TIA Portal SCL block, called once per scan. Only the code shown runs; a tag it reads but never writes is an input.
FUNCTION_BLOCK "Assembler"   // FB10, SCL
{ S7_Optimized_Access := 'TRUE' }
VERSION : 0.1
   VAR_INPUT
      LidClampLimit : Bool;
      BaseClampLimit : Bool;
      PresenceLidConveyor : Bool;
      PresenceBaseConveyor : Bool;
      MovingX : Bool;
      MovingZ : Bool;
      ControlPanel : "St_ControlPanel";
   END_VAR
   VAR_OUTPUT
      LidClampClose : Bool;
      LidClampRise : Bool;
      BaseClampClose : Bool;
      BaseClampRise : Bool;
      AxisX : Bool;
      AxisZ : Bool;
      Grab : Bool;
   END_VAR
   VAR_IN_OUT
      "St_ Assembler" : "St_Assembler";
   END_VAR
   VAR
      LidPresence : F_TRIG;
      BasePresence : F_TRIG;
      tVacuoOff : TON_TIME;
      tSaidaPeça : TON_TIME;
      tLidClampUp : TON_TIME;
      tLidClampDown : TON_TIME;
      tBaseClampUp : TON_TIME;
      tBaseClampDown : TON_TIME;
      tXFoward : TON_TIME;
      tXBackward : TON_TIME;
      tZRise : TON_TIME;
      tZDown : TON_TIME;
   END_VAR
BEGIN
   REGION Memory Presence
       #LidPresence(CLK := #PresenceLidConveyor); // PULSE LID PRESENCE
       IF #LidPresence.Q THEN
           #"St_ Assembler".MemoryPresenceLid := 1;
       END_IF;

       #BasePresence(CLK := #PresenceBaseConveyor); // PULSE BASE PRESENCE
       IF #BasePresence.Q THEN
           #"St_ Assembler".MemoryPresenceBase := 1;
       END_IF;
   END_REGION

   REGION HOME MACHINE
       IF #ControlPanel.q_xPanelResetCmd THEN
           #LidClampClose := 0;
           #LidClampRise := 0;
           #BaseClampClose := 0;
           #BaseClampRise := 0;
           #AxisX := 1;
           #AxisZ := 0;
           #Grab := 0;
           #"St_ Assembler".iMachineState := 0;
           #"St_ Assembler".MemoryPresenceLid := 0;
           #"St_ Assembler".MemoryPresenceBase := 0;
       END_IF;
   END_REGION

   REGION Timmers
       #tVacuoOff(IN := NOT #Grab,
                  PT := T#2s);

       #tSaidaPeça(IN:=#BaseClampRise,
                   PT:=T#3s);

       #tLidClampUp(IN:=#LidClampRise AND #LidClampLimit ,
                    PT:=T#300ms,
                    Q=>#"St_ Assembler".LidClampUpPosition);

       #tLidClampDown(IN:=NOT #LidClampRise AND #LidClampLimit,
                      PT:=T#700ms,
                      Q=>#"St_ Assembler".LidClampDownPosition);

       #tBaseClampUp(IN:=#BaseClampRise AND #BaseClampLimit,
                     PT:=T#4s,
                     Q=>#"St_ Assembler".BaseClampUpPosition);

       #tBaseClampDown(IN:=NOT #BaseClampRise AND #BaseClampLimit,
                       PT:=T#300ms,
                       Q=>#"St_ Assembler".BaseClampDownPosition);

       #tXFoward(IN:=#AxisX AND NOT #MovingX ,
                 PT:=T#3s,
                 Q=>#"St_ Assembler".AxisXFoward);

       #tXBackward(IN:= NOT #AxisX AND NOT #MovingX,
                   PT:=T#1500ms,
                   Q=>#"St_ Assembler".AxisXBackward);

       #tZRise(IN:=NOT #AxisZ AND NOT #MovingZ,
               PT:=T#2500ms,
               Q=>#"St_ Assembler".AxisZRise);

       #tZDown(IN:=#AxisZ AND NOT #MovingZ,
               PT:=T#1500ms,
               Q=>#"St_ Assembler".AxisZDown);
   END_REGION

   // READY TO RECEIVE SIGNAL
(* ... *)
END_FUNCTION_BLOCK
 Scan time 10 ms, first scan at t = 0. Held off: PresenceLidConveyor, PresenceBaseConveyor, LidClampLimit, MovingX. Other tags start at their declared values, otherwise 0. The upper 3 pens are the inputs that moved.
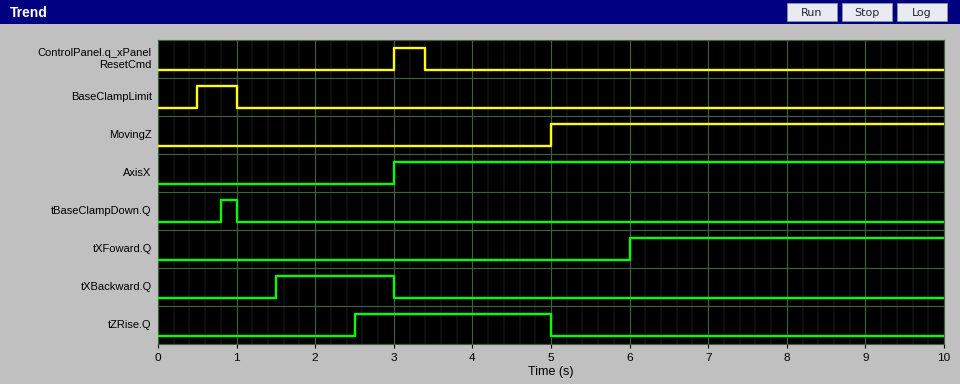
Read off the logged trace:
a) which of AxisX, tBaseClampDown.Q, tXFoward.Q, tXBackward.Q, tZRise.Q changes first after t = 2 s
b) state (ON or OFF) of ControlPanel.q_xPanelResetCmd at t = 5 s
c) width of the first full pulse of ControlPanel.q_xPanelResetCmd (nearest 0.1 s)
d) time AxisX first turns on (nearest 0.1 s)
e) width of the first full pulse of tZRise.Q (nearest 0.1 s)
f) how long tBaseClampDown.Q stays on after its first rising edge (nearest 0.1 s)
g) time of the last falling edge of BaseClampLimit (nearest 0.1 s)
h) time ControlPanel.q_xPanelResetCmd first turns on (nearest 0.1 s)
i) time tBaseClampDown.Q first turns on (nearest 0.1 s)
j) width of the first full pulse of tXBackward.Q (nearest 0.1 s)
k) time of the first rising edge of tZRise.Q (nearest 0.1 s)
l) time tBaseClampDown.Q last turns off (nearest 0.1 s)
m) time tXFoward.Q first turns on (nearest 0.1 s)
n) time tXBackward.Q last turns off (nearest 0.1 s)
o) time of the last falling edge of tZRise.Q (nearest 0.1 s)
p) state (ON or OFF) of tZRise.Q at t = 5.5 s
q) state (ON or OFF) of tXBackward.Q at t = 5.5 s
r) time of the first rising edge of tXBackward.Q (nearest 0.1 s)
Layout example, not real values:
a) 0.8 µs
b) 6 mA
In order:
a) tZRise.Q
b) OFF
c) 0.4 s
d) 3.0 s
e) 2.5 s
f) 0.2 s
g) 1.0 s
h) 3.0 s
i) 0.8 s
j) 1.5 s
k) 2.5 s
l) 1.0 s
m) 6.0 s
n) 3.0 s
o) 5.0 s
p) OFF
q) OFF
r) 1.5 s
